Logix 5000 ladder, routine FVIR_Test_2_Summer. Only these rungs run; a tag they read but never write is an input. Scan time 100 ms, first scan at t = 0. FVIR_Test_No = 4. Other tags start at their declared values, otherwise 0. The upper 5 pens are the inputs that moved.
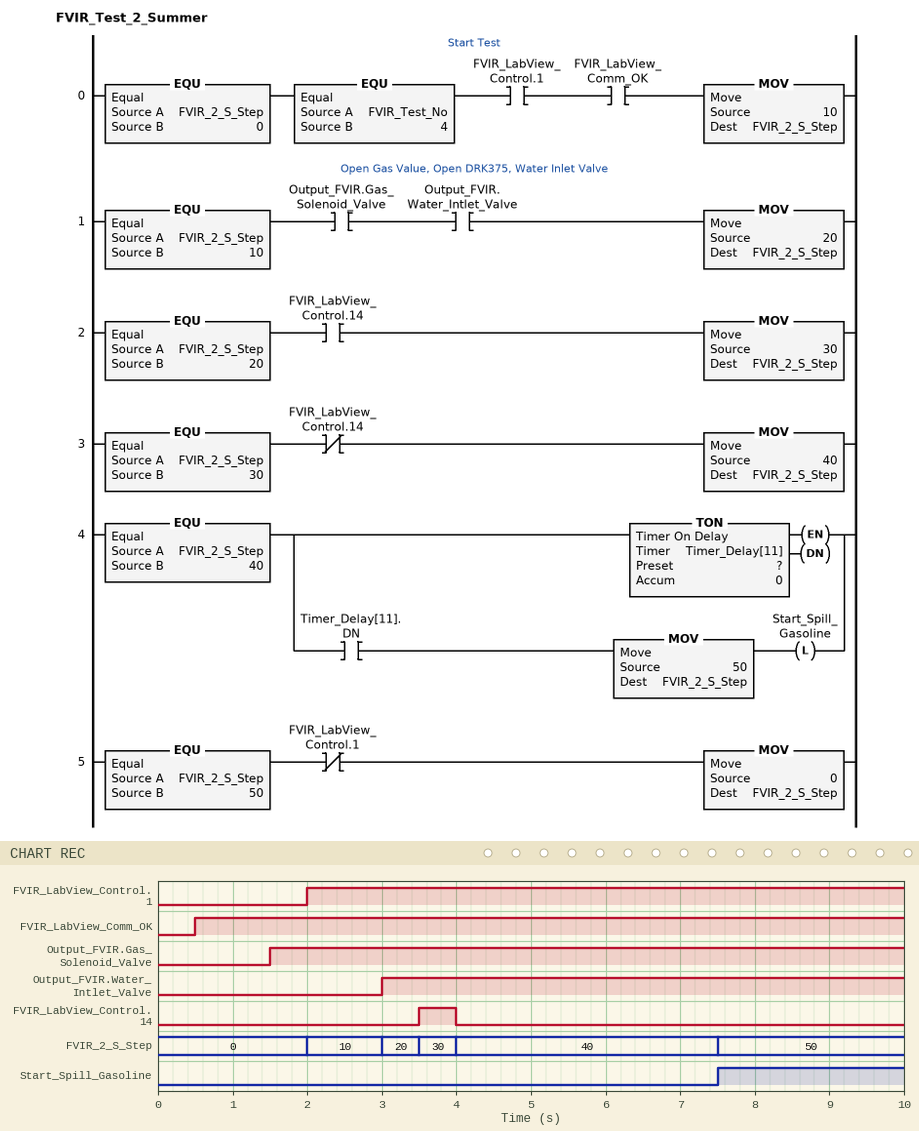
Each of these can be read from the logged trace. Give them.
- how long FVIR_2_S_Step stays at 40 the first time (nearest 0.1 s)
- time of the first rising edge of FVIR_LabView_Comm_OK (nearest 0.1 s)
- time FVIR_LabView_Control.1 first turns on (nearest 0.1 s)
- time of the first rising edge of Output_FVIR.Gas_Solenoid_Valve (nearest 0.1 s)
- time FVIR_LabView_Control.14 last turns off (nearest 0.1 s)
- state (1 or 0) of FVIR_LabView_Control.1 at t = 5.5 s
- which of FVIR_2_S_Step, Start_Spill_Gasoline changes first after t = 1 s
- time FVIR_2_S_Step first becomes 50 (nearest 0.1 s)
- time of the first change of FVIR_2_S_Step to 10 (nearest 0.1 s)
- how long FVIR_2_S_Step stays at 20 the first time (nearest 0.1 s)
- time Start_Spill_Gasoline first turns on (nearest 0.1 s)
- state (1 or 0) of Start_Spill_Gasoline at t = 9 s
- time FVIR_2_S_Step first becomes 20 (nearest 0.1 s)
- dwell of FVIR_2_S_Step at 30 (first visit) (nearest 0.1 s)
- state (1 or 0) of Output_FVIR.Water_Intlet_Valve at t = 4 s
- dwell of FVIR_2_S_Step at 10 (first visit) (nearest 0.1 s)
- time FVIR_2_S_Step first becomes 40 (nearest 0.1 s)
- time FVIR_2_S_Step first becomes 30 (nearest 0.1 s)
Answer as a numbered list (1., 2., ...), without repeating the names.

1. 3.5 s
2. 0.5 s
3. 2.0 s
4. 1.5 s
5. 4.0 s
6. 1
7. FVIR_2_S_Step
8. 7.5 s
9. 2.0 s
10. 0.5 s
11. 7.5 s
12. 1
13. 3.0 s
14. 0.5 s
15. 1
16. 1.0 s
17. 4.0 s
18. 3.5 s
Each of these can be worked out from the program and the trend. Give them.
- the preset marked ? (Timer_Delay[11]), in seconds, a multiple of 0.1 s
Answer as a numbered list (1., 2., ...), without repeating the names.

1. 3.5 s
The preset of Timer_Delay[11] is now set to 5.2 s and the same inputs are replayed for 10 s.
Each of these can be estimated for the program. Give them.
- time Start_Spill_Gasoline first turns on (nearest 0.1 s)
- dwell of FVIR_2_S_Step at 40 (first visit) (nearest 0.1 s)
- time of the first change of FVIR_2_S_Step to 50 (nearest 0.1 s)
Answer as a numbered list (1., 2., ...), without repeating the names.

1. 9.2 s
2. 5.2 s
3. 9.2 s
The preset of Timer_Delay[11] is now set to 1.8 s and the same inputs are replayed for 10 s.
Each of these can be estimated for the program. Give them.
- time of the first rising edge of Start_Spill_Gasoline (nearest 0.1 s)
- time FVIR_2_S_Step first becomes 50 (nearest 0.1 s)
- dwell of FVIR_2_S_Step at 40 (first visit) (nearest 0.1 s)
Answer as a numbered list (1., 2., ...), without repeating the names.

1. 5.8 s
2. 5.8 s
3. 1.8 s
